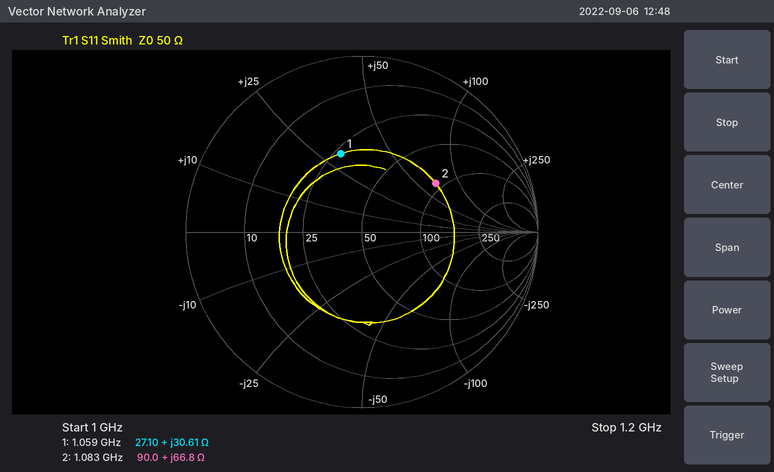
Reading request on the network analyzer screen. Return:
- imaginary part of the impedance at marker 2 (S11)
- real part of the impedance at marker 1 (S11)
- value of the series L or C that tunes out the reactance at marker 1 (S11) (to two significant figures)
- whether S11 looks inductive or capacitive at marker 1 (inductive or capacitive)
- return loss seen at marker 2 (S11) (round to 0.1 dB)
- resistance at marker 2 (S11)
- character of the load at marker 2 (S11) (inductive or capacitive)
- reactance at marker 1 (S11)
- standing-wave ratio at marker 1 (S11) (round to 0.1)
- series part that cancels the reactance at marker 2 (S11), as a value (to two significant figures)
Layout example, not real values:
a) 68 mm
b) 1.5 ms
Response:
a) +66.8 Ω
b) 27.10 Ω
c) 4.9 pF
d) inductive
e) 6.0 dB
f) 90.0 Ω
g) inductive
h) +30.61 Ω
i) 2.7
j) 2.2 pF
